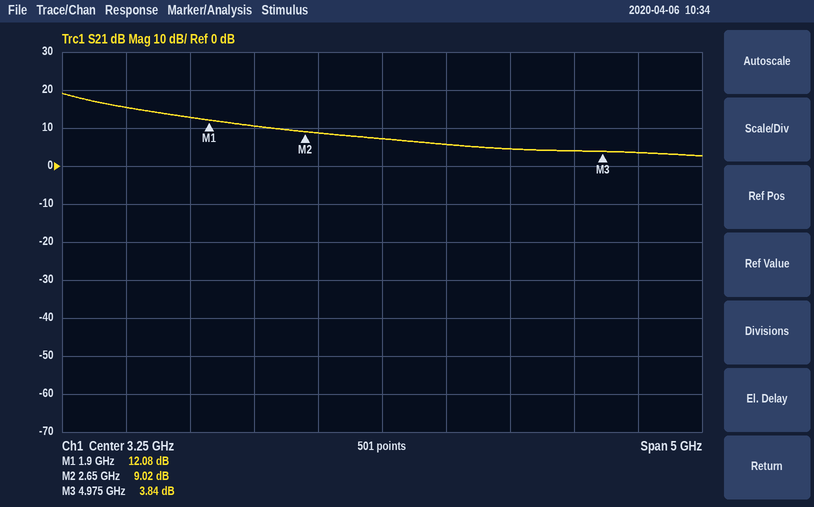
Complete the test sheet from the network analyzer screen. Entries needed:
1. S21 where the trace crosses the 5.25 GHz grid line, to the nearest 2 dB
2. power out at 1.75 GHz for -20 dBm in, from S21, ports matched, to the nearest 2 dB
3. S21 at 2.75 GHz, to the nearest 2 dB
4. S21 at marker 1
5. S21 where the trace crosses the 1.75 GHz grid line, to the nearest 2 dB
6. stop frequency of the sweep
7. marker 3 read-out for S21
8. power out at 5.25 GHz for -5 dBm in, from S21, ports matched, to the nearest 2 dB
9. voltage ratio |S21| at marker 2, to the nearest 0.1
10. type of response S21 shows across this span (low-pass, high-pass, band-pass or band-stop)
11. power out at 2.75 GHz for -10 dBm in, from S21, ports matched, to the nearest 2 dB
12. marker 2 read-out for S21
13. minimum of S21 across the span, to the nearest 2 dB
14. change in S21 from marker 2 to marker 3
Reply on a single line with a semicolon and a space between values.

4 dB; -8 dBm; 8 dB; 12.08 dB; 12 dB; 5.75 GHz; 3.84 dB; -2 dBm; 2.8; low-pass; -2 dBm; 9.02 dB; 2 dB; -5.18 dB
